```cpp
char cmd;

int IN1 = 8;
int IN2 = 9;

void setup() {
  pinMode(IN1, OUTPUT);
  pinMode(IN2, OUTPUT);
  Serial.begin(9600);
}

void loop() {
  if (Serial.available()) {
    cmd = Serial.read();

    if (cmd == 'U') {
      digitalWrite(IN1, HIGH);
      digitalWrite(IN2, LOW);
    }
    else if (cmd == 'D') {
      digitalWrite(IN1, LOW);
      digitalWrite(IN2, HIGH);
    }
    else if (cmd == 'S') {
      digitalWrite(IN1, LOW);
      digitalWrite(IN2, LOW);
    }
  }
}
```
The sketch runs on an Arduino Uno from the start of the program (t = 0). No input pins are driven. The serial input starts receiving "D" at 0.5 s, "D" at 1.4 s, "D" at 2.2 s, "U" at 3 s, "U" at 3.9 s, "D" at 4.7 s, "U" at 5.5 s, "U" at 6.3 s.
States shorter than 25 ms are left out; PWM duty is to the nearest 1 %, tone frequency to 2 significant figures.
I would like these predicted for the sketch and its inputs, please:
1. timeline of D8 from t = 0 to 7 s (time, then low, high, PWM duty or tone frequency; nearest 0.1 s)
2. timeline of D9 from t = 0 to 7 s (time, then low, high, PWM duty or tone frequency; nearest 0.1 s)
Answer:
0 s low; 3 s high; 4.7 s low; 5.5 s high
0 s low; 0.5 s high; 3 s low; 4.7 s high; 5.5 s low
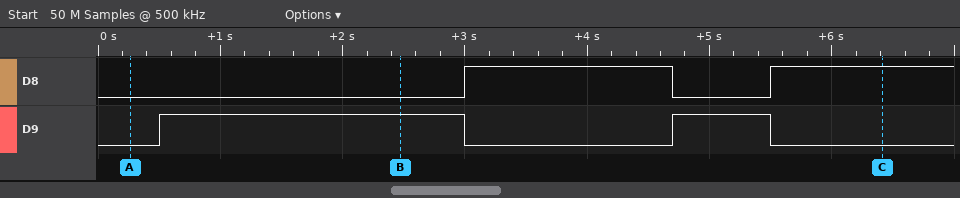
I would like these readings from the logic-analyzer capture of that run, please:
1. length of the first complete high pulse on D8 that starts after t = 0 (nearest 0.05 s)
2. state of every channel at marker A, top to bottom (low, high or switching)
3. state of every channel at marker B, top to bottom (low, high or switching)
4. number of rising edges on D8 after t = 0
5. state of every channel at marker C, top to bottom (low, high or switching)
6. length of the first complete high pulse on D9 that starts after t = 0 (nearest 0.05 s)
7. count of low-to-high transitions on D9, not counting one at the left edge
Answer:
1.70 s
D8 low, D9 low
D8 low, D9 high
2
D8 high, D9 low
2.50 s
2
